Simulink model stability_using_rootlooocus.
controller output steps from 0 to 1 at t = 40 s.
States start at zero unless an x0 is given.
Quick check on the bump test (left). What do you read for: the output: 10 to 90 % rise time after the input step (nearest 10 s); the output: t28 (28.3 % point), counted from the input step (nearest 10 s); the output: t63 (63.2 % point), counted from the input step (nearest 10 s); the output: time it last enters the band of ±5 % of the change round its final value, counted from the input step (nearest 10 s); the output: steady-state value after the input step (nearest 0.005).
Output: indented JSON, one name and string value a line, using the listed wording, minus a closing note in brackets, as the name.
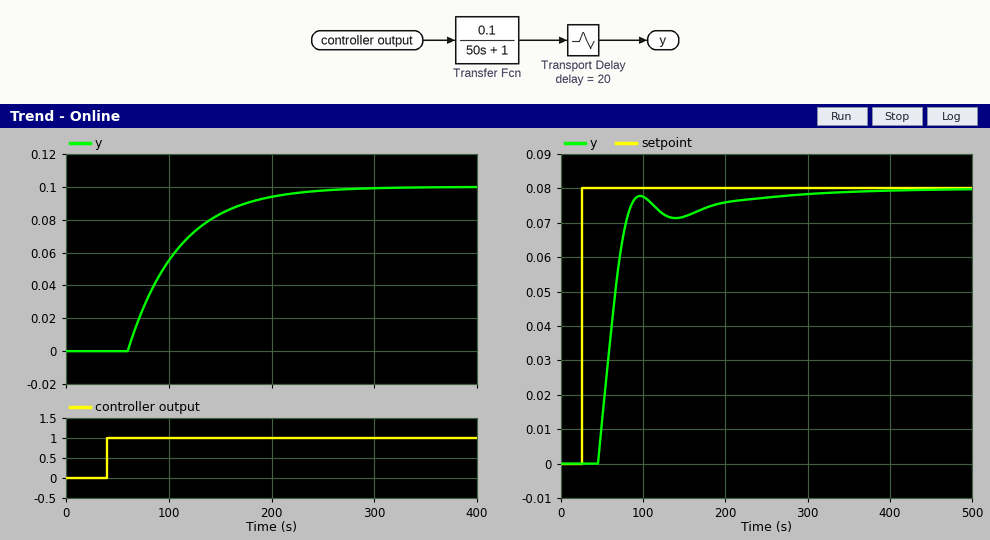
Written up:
{
  "the output: 10 to 90 % rise time after the input step": "110 s",
  "the output: t28 (28.3 % point), counted from the input step": "40 s",
  "the output: t63 (63.2 % point), counted from the input step": "70 s",
  "the output: time it last enters the band of ±5 % of the change round its final value, counted from the input step": "170 s",
  "the output: steady-state value after the input step": "0.100"
}
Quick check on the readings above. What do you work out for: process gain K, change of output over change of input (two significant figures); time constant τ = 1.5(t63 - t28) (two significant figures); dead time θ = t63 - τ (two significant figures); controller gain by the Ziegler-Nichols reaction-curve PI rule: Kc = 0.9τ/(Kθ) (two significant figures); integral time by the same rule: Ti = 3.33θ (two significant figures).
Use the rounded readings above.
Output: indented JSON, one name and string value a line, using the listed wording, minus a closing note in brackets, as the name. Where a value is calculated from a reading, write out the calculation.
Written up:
{
  "process gain K, change of output over change of input": "(0.1 - 0) / 1 = 0.10",
  "time constant τ = 1.5(t63 - t28)": "1.5 × (70 - 40) = 45 s",
  "dead time θ = t63 - τ": "70 - 45 = 25 s",
  "controller gain by the Ziegler-Nichols reaction-curve PI rule: Kc = 0.9τ/(Kθ)": "0.9 × 45 / (0.1 × 25) = 16",
  "integral time by the same rule: Ti = 3.33θ": "3.33 × 25 = 83 s"
}
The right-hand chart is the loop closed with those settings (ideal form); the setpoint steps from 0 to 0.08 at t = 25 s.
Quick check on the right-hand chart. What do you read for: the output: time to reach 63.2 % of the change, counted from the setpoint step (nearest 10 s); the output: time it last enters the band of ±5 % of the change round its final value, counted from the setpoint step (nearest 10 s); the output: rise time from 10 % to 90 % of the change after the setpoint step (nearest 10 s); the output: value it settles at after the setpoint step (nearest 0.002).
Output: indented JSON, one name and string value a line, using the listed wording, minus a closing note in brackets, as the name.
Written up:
{
  "the output: time to reach 63.2 % of the change, counted from the setpoint step": "40 s",
  "the output: time it last enters the band of ±5 % of the change round its final value, counted from the setpoint step": "180 s",
  "the output: rise time from 10 % to 90 % of the change after the setpoint step": "30 s",
  "the output: value it settles at after the setpoint step": "0.080"
}
